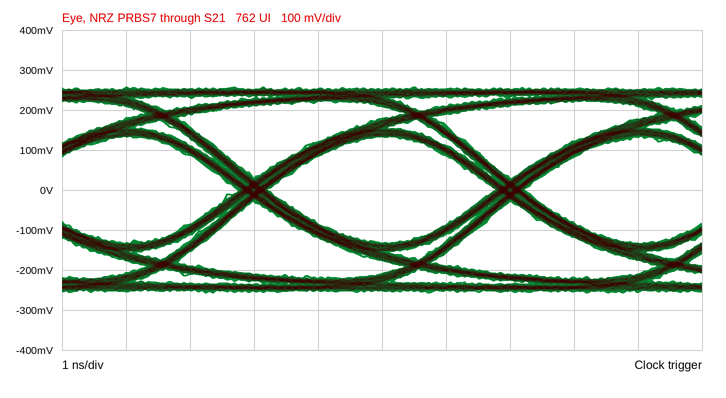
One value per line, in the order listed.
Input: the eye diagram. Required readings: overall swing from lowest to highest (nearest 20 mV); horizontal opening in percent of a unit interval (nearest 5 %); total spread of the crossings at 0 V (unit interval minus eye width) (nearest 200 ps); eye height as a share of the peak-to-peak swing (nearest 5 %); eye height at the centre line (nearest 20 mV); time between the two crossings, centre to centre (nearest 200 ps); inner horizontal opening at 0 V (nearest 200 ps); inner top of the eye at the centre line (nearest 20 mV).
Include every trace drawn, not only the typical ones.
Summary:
520 mV
90 %
400 ps
50 %
260 mV
4.0 ns
3.6 ns
140 mV
